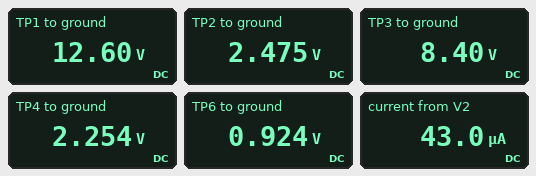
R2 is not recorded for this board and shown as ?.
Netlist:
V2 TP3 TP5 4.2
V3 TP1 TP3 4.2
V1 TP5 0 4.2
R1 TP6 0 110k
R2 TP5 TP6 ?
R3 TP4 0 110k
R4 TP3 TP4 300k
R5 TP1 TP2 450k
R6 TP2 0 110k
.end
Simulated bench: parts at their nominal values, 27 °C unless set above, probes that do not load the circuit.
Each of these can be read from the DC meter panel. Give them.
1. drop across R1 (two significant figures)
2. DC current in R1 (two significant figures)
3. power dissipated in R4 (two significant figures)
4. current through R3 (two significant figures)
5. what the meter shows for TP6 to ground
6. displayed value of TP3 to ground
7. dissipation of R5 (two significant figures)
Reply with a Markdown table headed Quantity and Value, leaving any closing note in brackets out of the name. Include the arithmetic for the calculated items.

| Quantity | Value |
|---|---|
| drop across R1 | 924 mV = 920 mV |
| DC current in R1 | (924 mV) / 110 kΩ = 8.4 µA |
| power dissipated in R4 | (8.4 V - 2.254 V)^2 / 300 kΩ = 130 µW |
| current through R3 | (2.254 V) / 110 kΩ = 20 µA |
| what the meter shows for TP6 to ground | 0.924 V |
| displayed value of TP3 to ground | 8.40 V |
| dissipation of R5 | (12.6 V - 2.475 V)^2 / 450 kΩ = 230 µW |
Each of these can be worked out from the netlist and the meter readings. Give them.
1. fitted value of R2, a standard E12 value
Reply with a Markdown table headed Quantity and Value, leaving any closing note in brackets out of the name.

| Quantity | Value |
|---|---|
| fitted value of R2, a standard E12 value | 390 kΩ |
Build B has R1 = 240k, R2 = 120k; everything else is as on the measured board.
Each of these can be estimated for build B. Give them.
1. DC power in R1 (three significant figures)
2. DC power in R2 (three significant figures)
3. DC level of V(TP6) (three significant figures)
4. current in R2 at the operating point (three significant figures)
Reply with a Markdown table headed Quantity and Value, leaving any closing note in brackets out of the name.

| Quantity | Value |
|---|---|
| DC power in R1 | 32.7 µW |
| DC power in R2 | 16.3 µW |
| DC level of V(TP6) | 2.80 V |
| current in R2 at the operating point | 11.7 µA |
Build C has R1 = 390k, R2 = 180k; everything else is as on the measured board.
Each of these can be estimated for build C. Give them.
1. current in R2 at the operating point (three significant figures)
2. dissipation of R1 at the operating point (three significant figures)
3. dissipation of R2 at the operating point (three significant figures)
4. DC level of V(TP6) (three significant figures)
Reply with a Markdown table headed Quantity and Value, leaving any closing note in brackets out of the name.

| Quantity | Value |
|---|---|
| current in R2 at the operating point | 7.37 µA |
| dissipation of R1 at the operating point | 21.2 µW |
| dissipation of R2 at the operating point | 9.77 µW |
| DC level of V(TP6) | 2.87 V |
